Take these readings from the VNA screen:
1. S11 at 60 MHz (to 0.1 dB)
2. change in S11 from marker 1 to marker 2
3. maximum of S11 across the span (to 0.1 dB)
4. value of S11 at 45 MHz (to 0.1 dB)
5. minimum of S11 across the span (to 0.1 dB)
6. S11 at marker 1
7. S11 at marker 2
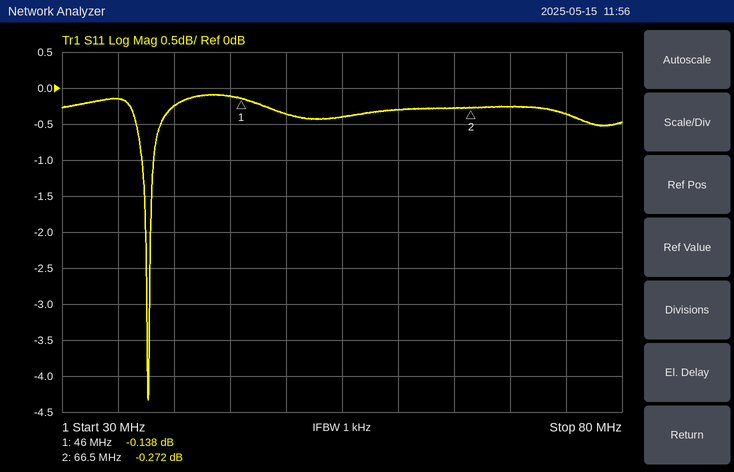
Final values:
-0.3 dB
-0.134 dB
-0.1 dB
-0.1 dB
-4.3 dB
-0.138 dB
-0.272 dB
